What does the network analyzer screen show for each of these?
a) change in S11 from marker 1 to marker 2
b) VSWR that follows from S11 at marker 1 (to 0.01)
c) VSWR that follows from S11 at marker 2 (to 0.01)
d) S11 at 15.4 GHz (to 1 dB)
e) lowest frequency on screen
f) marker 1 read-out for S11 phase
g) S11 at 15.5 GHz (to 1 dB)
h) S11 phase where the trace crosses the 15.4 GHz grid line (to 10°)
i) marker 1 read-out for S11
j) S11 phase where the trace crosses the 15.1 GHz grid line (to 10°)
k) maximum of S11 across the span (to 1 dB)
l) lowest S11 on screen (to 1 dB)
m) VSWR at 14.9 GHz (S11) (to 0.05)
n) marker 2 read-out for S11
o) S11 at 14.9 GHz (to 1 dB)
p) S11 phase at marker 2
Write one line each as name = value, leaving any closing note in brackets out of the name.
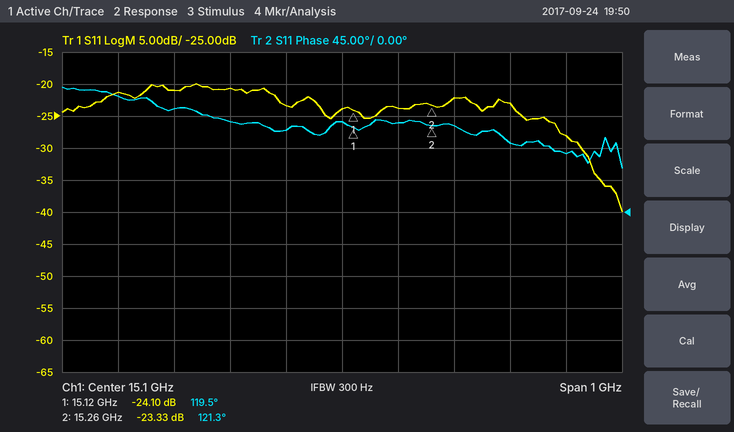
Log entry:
change in S11 from marker 1 to marker 2 = 0.77 dB
VSWR that follows from S11 at marker 1 = 1.13
VSWR that follows from S11 at marker 2 = 1.15
S11 at 15.4 GHz = -23 dB
lowest frequency on screen = 14.6 GHz
marker 1 read-out for S11 phase = 119.5°
S11 at 15.5 GHz = -28 dB
S11 phase where the trace crosses the 15.4 GHz grid line = 100°
marker 1 read-out for S11 = -24.10 dB
S11 phase where the trace crosses the 15.1 GHz grid line = 130°
maximum of S11 across the span = -20 dB
lowest S11 on screen = -40 dB
VSWR at 14.9 GHz (S11) = 1.20
marker 2 read-out for S11 = -23.33 dB
S11 at 14.9 GHz = -21 dB
S11 phase at marker 2 = 121.3°
